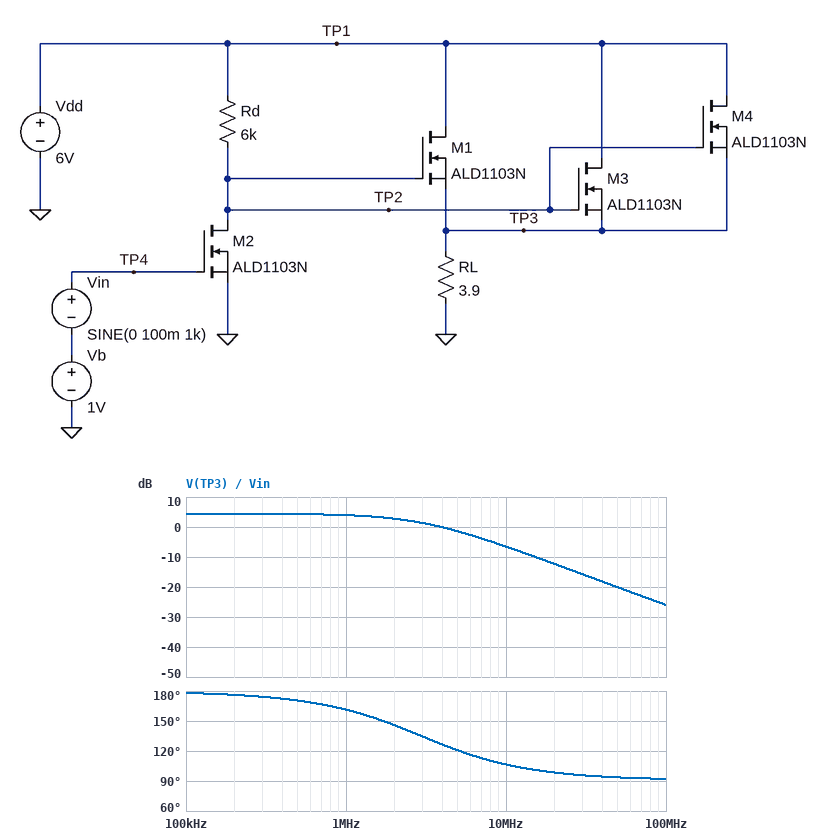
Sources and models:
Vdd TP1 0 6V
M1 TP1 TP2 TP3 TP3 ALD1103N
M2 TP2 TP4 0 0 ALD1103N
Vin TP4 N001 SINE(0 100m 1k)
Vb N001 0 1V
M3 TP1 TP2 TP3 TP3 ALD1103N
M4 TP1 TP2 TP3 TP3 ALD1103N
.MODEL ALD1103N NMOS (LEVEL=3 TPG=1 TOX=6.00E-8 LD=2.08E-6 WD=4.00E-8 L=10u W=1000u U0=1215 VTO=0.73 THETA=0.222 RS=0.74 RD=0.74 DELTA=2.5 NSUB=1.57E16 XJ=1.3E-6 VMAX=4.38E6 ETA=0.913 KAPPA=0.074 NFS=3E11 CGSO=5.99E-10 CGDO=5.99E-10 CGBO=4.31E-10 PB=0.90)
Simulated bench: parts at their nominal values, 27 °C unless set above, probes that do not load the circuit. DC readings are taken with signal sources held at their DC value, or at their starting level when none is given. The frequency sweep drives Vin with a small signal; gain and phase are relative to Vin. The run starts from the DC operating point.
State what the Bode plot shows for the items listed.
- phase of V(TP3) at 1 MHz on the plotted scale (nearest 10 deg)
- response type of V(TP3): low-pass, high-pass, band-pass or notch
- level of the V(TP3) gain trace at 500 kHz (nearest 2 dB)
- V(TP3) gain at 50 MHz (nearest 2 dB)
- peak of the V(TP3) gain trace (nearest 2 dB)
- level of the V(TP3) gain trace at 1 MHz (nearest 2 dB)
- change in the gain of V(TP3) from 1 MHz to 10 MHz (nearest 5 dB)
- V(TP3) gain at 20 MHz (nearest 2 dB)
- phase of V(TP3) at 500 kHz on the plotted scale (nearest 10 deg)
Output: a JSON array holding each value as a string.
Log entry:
["160 deg", "low-pass", "4 dB", "-20 dB", "4 dB", "4 dB", "-10 dB", "-12 dB", "170 deg"]
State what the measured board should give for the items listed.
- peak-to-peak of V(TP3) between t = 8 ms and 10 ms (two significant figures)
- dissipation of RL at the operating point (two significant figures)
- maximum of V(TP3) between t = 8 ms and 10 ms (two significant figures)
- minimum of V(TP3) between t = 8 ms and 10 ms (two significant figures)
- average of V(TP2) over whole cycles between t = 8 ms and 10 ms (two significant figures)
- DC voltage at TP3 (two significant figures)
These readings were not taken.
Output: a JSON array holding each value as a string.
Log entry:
["310 mV", "9.3 mW", "350 mV", "39 mV", "3.2 V", "190 mV"]
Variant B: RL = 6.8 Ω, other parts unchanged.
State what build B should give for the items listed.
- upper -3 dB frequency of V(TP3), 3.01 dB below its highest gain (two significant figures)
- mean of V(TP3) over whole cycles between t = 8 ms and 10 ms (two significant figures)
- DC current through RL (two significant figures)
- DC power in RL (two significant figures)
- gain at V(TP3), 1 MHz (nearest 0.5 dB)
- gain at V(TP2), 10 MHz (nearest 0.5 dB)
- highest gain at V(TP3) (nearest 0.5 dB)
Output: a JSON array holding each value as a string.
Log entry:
["3.1 MHz", "310 mV", "45 mA", "14 mW", "8.0 dB", "12.5 dB", "8.5 dB"]
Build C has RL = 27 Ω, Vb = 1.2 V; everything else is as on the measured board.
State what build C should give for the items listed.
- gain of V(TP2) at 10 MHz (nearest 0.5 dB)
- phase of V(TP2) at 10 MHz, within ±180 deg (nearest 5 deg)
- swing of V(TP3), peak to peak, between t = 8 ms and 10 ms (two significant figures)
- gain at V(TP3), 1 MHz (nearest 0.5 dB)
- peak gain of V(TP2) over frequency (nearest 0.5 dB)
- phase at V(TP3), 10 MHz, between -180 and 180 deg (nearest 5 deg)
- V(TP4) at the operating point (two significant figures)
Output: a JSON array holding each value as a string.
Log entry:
["2.5 dB", "155 deg", "190 mV", "-54.0 dB", "3.0 dB", "-115 deg", "1.2 V"]
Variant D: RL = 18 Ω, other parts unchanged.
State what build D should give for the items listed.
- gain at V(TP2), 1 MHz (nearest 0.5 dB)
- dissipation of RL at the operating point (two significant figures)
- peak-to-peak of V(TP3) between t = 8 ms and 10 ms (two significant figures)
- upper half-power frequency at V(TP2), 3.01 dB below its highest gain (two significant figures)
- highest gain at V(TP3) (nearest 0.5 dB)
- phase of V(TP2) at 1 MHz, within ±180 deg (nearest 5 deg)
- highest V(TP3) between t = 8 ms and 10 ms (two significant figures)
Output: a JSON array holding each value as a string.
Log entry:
["23.0 dB", "22 mW", "960 mV", "3.7 MHz", "14.0 dB", "165 deg", "1.1 V"]
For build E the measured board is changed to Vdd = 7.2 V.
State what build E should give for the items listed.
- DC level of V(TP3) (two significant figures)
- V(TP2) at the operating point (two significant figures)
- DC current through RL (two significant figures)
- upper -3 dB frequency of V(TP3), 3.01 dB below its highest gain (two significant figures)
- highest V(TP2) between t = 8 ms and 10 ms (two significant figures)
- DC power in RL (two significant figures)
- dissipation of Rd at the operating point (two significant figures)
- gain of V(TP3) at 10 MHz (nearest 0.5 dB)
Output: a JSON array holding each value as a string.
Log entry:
["330 mV", "4.3 V", "84 mA", "3.0 MHz", "5.6 V", "27 mW", "1.4 mW", "-5.0 dB"]
